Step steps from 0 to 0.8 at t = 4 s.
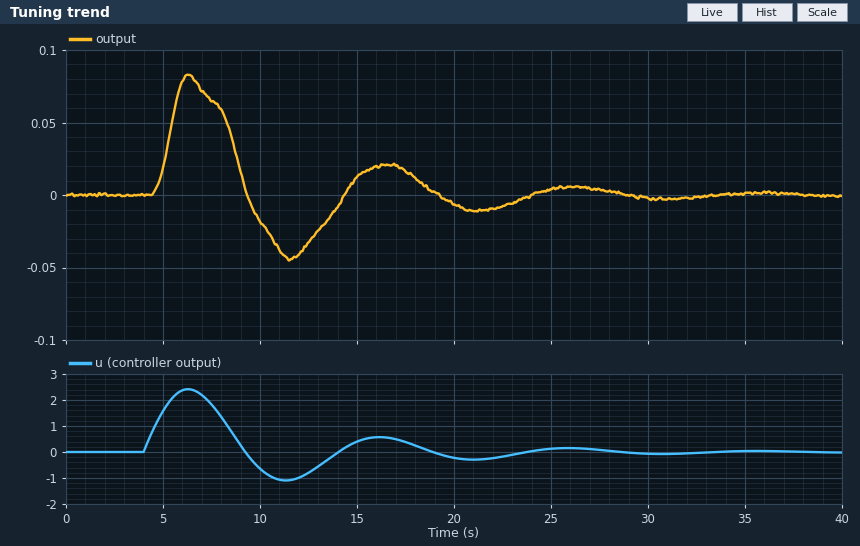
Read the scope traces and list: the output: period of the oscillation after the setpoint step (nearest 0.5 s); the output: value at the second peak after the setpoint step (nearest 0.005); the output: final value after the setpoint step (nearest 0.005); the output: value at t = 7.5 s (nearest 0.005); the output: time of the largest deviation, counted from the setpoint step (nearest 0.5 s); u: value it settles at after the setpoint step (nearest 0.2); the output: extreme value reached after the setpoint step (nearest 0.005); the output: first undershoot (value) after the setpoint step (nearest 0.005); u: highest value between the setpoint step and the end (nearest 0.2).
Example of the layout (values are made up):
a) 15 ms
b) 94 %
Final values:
a) 10.5 s
b) 0.020
c) 0.000
d) 0.065
e) 2.5 s
f) 0.0
g) 0.085
h) -0.045
i) 2.4
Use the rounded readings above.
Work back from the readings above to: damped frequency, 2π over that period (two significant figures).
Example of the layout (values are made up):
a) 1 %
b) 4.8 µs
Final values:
a) 0.60 rad/s
